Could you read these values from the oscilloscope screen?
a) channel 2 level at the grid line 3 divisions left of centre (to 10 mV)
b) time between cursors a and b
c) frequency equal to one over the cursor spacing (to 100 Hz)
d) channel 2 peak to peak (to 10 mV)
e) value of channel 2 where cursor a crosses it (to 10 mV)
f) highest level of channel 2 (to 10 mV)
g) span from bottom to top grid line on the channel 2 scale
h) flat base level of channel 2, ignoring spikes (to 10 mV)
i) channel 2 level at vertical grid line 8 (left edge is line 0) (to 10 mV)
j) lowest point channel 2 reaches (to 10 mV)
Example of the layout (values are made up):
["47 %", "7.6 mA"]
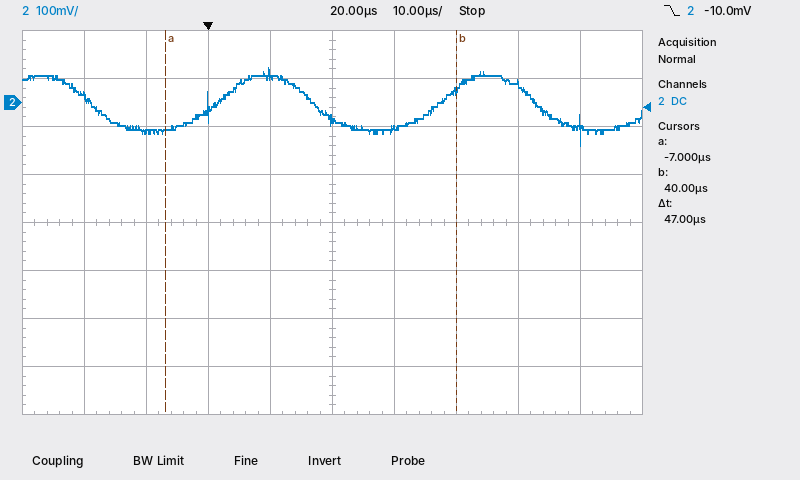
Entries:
["-60 mV", "47 µs", "21.3 kHz", "160 mV", "-60 mV", "70 mV", "800 mV", "-60 mV", "40 mV", "-90 mV"]
